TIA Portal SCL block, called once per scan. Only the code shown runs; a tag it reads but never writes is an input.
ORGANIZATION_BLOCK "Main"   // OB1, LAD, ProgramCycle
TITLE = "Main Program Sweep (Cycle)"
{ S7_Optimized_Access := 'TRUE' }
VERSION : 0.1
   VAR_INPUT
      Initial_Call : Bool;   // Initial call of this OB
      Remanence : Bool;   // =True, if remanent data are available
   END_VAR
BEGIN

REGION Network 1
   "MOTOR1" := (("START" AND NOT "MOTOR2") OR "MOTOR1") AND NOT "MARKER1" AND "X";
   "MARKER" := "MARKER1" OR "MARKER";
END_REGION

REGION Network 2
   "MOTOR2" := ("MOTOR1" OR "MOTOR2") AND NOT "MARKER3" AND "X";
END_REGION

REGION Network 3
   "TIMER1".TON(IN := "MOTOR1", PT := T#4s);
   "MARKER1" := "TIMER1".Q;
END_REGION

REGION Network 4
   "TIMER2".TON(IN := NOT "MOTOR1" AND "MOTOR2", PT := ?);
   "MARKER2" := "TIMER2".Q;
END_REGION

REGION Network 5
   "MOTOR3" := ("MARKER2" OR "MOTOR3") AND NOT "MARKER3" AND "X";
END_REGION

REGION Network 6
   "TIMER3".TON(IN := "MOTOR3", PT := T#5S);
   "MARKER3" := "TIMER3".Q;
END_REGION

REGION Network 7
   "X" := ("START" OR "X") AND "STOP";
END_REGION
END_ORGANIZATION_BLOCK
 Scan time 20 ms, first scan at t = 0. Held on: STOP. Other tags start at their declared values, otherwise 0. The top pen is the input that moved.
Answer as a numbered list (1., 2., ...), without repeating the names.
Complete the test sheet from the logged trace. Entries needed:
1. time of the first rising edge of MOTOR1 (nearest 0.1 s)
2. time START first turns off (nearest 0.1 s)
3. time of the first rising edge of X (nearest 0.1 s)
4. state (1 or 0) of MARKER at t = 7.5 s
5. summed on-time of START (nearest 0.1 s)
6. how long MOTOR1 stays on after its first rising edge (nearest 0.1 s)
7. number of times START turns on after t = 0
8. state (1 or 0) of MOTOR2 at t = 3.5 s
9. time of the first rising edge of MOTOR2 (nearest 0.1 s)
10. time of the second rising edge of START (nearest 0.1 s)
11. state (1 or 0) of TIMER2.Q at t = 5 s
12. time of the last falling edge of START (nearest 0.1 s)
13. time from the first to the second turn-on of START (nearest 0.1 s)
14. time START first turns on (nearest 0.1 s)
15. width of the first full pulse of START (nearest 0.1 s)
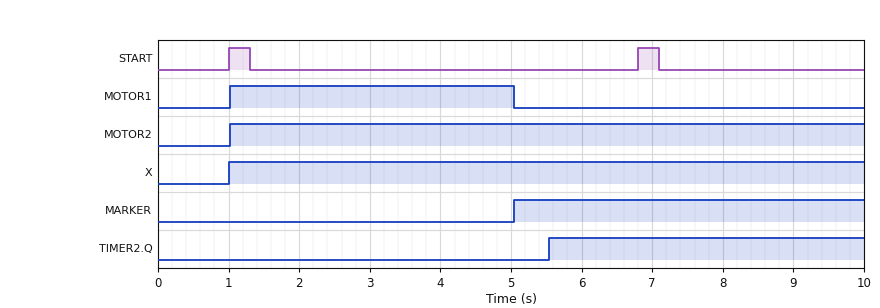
1. 1.0 s
2. 1.3 s
3. 1.0 s
4. 1
5. 0.6 s
6. 4.0 s
7. 2
8. 1
9. 1.0 s
10. 6.8 s
11. 0
12. 7.1 s
13. 5.8 s
14. 1.0 s
15. 0.3 s
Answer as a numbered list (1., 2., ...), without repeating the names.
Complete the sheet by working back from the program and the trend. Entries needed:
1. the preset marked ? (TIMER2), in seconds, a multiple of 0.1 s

1. 0.5 s
